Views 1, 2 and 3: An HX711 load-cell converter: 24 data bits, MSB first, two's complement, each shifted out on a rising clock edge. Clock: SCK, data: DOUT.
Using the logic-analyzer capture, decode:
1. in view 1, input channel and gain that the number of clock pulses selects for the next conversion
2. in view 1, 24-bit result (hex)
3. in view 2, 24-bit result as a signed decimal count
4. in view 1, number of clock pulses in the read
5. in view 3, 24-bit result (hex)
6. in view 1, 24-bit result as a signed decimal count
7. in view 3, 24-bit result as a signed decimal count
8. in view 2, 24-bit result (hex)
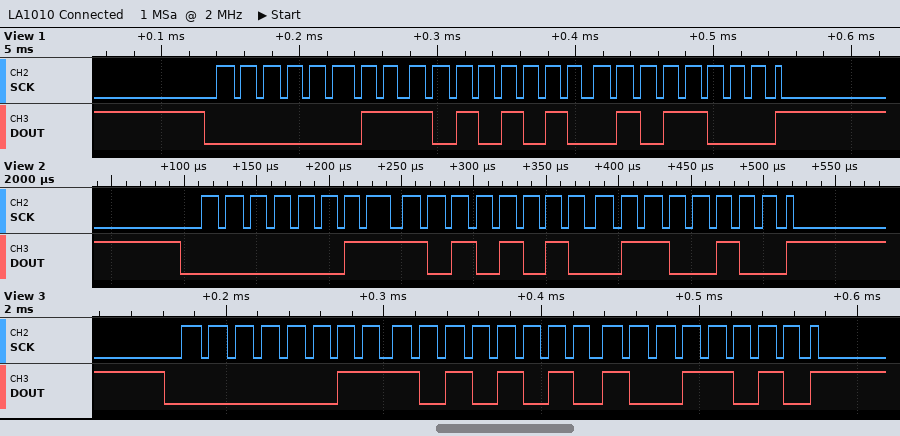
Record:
channel A, gain 128
0x03AA58
240228
25
0x03AA9A
240216
240282
0x03AA64
